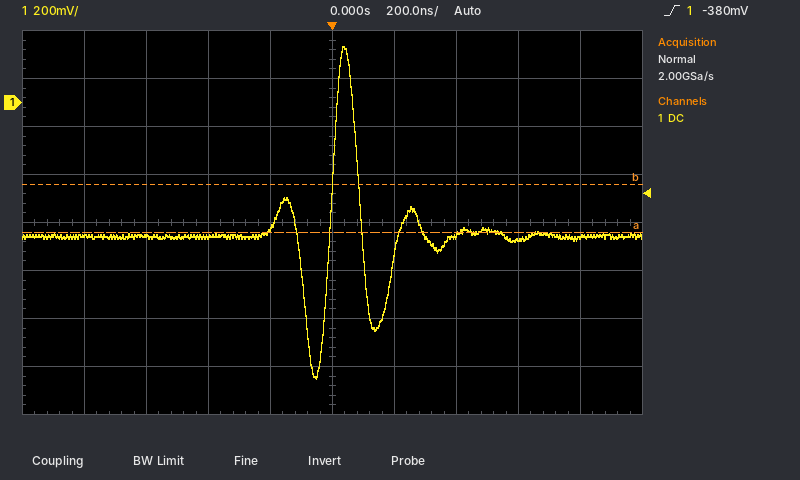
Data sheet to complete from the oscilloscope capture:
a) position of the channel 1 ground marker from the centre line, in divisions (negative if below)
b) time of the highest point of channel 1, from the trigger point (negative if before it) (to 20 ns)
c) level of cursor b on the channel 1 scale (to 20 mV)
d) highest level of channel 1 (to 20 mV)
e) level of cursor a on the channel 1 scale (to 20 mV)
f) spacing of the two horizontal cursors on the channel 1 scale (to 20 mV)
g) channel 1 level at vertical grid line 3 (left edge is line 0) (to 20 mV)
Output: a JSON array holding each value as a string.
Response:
["+2.5 div", "+40 ns", "-340 mV", "240 mV", "-540 mV", "200 mV", "-560 mV"]
